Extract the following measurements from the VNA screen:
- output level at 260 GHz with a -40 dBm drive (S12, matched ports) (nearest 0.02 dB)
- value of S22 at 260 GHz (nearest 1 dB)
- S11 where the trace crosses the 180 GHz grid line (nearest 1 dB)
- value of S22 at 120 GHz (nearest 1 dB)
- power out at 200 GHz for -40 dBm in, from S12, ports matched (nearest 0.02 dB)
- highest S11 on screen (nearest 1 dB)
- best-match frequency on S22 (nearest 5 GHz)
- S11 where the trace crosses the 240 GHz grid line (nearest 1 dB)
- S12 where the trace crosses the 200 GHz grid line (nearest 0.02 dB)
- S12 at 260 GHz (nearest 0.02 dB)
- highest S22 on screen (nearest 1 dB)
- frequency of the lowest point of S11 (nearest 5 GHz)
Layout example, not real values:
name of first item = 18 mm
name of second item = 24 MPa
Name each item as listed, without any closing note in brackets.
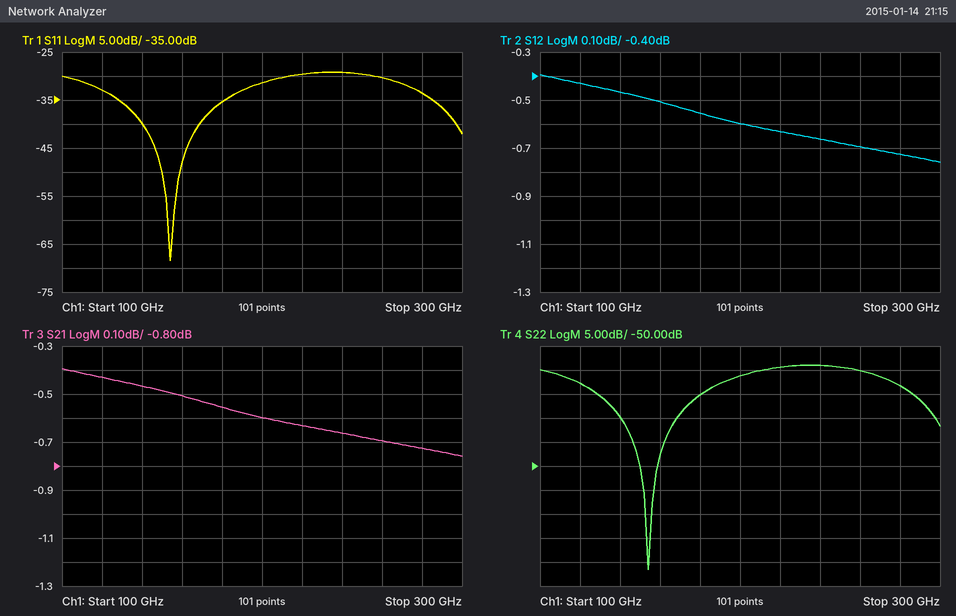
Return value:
output level at 260 GHz with a -40 dBm drive (S12, matched ports) = -40.70 dBm
value of S22 at 260 GHz = -30 dB
S11 where the trace crosses the 180 GHz grid line = -35 dB
value of S22 at 120 GHz = -33 dB
power out at 200 GHz for -40 dBm in, from S12, ports matched = -40.60 dBm
highest S11 on screen = -29 dB
best-match frequency on S22 = 155 GHz
S11 where the trace crosses the 240 GHz grid line = -29 dB
S12 where the trace crosses the 200 GHz grid line = -0.60 dB
S12 at 260 GHz = -0.70 dB
highest S22 on screen = -29 dB
frequency of the lowest point of S11 = 155 GHz
